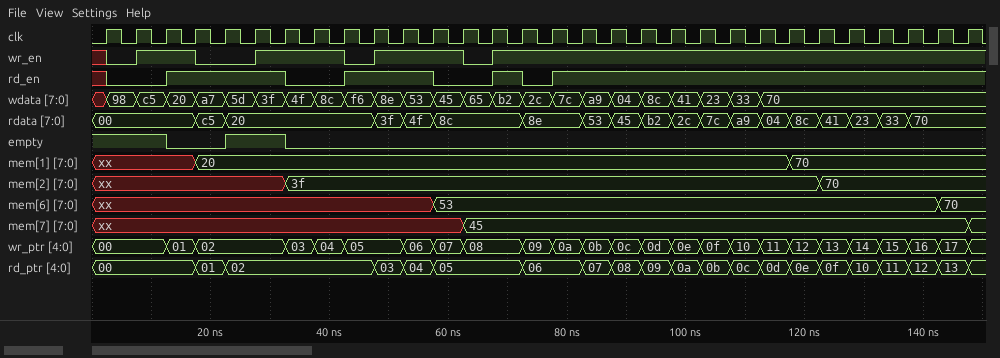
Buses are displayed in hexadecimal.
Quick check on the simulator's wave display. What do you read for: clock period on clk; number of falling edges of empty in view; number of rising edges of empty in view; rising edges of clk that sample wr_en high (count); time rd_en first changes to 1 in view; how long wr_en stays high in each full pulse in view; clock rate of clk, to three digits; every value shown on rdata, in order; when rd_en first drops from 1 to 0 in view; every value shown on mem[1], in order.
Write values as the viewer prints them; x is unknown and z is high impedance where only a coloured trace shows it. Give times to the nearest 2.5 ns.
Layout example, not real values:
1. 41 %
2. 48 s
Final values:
1. 5 ns
2. 2
3. 1
4. 24
5. 12.5 ns
6. 10 ns, 15 ns, 15 ns
7. 200 MHz
8. 00, c5, 20, 3f, 4f, 8c, 8e, 53, 45, b2, 2c, 7c, a9, 04, 8c, 41, 23, 33, 70
9. 32.5 ns
10. xx, 20, 70
